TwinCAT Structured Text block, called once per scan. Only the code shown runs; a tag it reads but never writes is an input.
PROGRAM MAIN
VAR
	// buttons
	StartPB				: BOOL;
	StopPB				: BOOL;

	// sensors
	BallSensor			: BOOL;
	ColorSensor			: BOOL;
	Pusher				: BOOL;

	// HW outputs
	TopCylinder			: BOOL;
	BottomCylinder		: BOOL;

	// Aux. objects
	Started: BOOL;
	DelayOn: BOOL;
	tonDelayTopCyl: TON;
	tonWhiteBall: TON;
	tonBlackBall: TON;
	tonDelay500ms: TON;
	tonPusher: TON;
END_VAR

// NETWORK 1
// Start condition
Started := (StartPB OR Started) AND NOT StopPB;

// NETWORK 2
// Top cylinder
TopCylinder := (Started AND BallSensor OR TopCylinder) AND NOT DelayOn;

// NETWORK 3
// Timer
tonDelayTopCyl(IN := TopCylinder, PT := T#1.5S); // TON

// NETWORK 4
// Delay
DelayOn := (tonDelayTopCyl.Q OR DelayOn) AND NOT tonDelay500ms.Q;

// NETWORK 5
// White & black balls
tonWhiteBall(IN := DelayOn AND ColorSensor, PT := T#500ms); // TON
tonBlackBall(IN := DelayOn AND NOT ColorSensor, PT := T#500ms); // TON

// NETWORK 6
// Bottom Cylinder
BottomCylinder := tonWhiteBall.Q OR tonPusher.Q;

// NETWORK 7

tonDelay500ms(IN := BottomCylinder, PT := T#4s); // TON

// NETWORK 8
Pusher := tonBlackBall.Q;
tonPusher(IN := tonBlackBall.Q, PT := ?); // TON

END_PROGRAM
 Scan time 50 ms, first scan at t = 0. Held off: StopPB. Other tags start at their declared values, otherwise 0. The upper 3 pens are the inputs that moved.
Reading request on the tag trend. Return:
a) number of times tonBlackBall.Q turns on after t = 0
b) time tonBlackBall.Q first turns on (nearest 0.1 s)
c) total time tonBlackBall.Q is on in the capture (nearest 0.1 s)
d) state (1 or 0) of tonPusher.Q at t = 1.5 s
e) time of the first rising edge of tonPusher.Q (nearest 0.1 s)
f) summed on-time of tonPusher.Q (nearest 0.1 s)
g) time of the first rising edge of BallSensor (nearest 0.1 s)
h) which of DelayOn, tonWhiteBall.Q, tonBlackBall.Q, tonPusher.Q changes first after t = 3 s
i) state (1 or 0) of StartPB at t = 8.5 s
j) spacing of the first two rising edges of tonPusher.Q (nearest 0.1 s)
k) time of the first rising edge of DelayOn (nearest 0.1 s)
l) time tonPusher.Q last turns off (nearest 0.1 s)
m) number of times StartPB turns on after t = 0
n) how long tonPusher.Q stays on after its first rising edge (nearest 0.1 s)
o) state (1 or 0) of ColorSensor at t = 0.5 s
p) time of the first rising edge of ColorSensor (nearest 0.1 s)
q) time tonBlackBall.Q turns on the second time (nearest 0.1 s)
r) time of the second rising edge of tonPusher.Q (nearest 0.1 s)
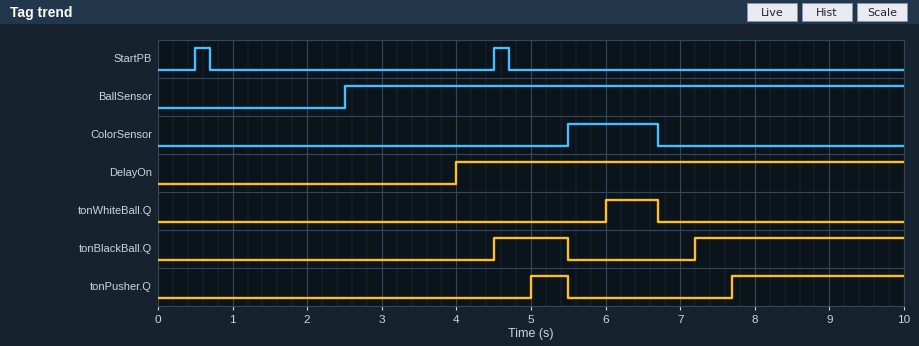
2
4.5 s
3.8 s
0
5.0 s
2.8 s
2.5 s
DelayOn
0
2.7 s
4.0 s
5.5 s
2
0.5 s
0
5.5 s
7.2 s
7.7 s
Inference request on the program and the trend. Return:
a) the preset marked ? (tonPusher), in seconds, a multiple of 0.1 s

0.5 s
